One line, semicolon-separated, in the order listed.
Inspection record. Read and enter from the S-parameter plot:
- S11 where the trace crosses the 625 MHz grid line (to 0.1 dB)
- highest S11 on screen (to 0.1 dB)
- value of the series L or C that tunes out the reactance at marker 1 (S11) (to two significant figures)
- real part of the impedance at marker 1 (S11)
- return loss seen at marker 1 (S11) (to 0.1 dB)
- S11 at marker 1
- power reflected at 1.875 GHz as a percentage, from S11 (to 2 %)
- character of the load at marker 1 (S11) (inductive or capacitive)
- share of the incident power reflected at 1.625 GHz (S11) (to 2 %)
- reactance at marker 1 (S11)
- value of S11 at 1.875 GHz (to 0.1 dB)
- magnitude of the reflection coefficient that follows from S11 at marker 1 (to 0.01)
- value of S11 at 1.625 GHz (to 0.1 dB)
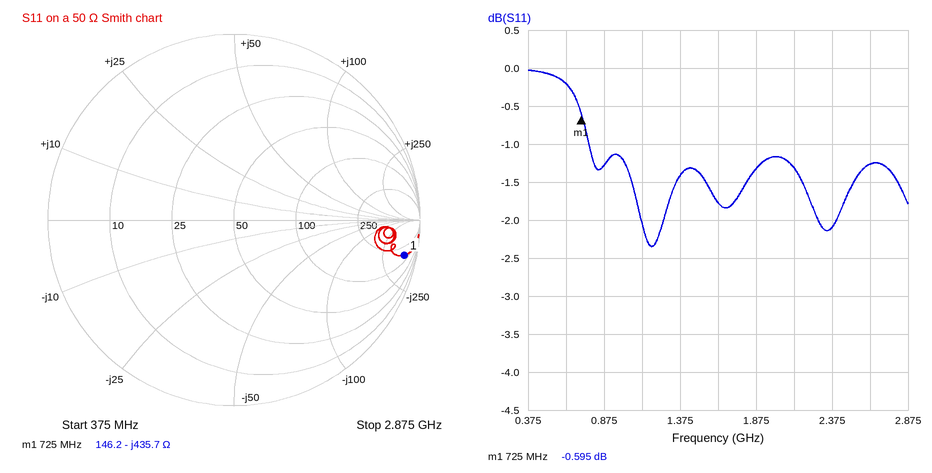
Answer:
-0.2 dB; 0.0 dB; 96 nH; 146.2 Ω; 0.6 dB; -0.595 dB; 74 %; capacitive; 66 %; -435.7 Ω; -1.3 dB; 0.93; -1.8 dB
